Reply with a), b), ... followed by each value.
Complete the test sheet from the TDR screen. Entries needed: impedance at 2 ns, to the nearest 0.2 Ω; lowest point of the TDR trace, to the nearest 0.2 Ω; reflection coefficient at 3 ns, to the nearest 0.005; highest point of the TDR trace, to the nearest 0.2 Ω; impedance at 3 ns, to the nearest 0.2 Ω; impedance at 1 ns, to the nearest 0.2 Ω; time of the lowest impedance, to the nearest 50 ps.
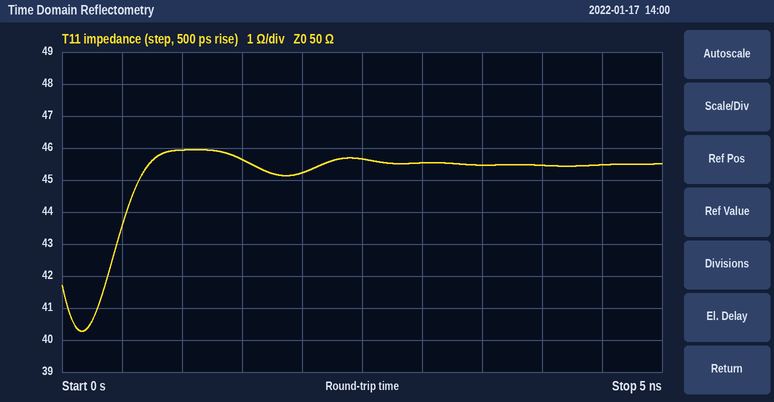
a) 45.2 Ω
b) 40.2 Ω
c) -0.045
d) 46.0 Ω
e) 45.6 Ω
f) 46.0 Ω
g) 150 ps
